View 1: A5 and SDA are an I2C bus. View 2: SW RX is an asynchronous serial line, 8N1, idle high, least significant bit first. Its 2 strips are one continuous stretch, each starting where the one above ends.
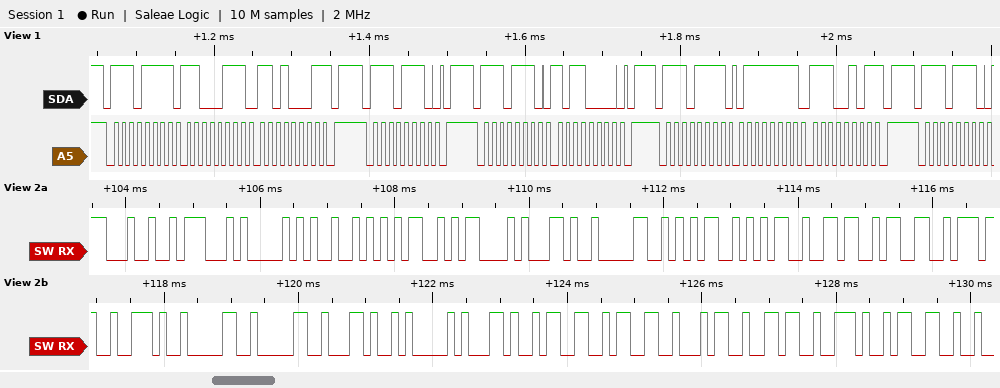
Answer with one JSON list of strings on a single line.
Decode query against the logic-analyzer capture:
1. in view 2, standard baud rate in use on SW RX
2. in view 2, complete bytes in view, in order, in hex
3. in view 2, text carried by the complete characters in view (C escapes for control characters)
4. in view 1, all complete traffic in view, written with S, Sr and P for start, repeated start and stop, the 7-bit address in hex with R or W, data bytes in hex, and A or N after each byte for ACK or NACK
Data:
["9600 baud", "24 47 50 52 4D 43 2C 30 35 35 36 33 37 2E 30 30 2C 41 2C 33 33 34 36 2E 33", "\"$GPRMC,055637.00,A,3346.3\"", "S 77R A C7 A D1 N P S 77W A P S 77W A B0 A P S 77R A 7F A E5 N P S 77W A"]
